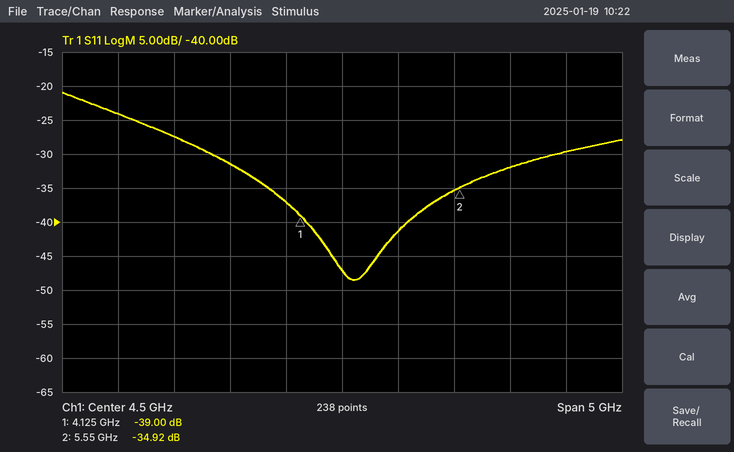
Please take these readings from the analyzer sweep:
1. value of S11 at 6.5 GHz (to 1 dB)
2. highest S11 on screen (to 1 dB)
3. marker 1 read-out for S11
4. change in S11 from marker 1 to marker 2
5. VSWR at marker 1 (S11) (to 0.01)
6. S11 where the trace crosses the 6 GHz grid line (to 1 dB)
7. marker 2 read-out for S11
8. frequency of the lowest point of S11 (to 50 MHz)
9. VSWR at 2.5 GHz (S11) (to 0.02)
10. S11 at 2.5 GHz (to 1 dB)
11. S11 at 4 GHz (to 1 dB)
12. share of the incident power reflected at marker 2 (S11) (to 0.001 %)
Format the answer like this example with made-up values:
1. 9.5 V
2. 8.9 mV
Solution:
1. -30 dB
2. -21 dB
3. -39.00 dB
4. 4.08 dB
5. 1.02
6. -32 dB
7. -34.92 dB
8. 4.60 GHz
9. 1.14
10. -24 dB
11. -37 dB
12. 0.032 %
